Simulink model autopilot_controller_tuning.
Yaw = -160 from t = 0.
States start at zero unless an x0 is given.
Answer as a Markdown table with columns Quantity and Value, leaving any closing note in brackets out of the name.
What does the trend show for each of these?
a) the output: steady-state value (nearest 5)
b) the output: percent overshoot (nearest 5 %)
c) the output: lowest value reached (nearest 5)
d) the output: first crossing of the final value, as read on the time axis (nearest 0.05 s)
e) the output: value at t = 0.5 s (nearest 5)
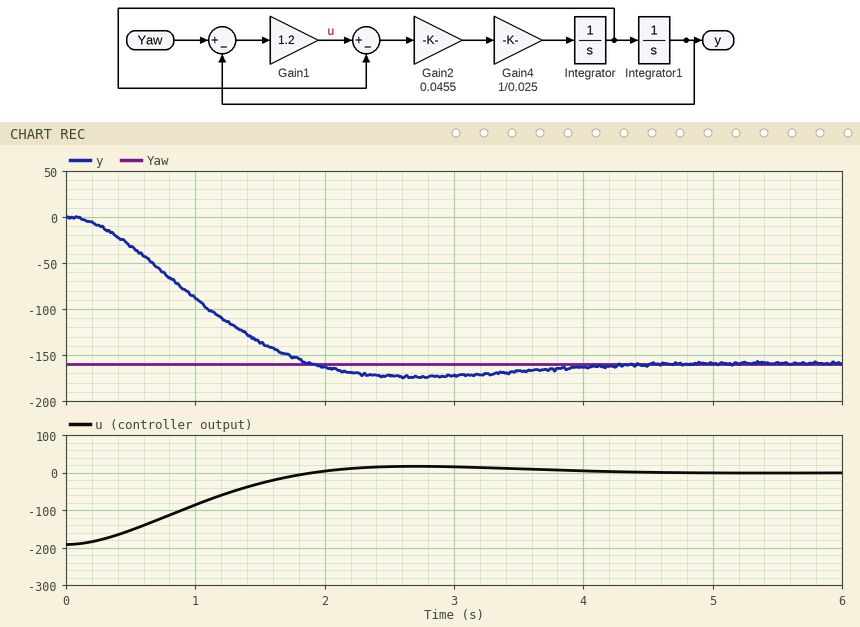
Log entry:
| Quantity | Value |
|---|---|
| the output: steady-state value | -160 |
| the output: percent overshoot | 10 % |
| the output: lowest value reached | -175 |
| the output: first crossing of the final value, as read on the time axis | 1.90 s |
| the output: value at t = 0.5 s | -30 |
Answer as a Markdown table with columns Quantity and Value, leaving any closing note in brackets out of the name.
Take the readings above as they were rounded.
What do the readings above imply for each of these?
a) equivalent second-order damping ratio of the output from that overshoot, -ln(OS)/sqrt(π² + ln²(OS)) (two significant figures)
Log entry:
| Quantity | Value |
|---|---|
| equivalent second-order damping ratio of the output from that overshoot, -ln(OS)/sqrt(π² + ln²(OS)) | 0.59 |
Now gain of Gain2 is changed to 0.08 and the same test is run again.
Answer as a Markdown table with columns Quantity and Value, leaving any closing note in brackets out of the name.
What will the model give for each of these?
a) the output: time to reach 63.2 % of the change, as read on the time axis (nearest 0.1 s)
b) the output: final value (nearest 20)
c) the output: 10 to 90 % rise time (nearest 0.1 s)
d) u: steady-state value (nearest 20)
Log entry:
| Quantity | Value |
|---|---|
| the output: time to reach 63.2 % of the change, as read on the time axis | 1.0 s |
| the output: final value | -160 |
| the output: 10 to 90 % rise time | 1.3 s |
| u: steady-state value | 0 |
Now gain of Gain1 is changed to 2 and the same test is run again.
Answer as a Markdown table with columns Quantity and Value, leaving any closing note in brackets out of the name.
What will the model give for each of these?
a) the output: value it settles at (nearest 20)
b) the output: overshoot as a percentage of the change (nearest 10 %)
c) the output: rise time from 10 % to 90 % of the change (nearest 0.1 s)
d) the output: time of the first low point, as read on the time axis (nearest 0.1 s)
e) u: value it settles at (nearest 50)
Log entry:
| Quantity | Value |
|---|---|
| the output: value it settles at | -160 |
| the output: overshoot as a percentage of the change | 20 % |
| the output: rise time from 10 % to 90 % of the change | 0.8 s |
| the output: time of the first low point, as read on the time axis | 1.9 s |
| u: value it settles at | 0 |
